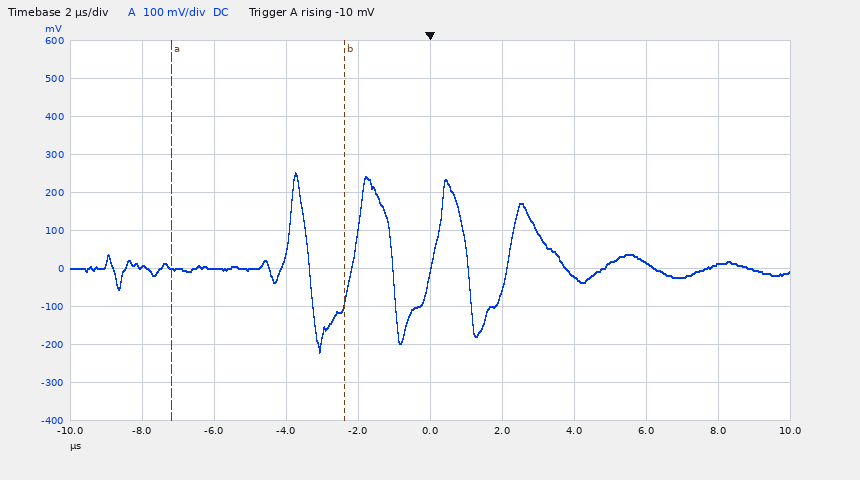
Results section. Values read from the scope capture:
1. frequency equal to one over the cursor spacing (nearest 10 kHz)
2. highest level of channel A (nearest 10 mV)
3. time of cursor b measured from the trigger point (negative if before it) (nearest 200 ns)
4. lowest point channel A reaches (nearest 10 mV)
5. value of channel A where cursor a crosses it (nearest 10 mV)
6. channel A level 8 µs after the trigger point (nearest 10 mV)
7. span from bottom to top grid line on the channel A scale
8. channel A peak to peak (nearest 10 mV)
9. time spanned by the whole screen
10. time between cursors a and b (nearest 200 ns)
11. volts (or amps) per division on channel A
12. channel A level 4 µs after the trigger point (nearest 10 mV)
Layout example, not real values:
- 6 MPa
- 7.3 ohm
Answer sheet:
- 210 kHz
- 250 mV
- -2.4 µs
- -220 mV
- 0 mV
- 10 mV
- 1 V
- 470 mV
- 20 µs
- 4.8 µs
- 100 mV
- -20 mV
